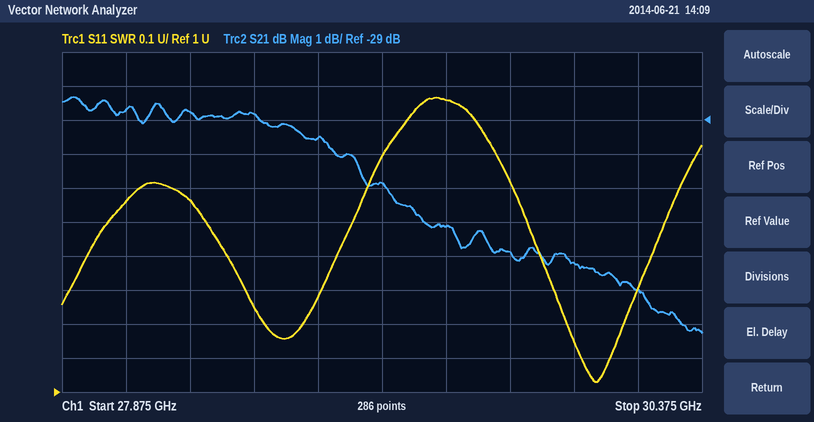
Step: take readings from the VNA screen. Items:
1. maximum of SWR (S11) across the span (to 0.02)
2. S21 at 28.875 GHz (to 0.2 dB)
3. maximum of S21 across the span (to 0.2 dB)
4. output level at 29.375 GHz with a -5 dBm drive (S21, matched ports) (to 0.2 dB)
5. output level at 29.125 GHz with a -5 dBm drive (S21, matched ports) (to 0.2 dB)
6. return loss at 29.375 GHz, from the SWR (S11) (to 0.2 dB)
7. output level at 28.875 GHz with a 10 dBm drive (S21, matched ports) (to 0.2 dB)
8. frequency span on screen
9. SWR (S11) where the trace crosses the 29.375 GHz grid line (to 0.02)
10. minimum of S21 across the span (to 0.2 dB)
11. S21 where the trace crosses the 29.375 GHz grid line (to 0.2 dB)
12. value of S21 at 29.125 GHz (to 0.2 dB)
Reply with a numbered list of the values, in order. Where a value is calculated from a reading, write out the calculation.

1. 1.86
2. -29.6 dB
3. -28.4 dB
4. -5 dBm + (-32.2 dB) = -37.2 dBm
5. -5 dBm + (-30.8 dB) = -35.8 dBm
6. −20 log10((1.86 − 1)/(1.86 + 1)) ≈ 10.4 dB
7. 10 dBm + (-29.6 dB) = -19.6 dBm
8. 2.5 GHz
9. 1.86
10. -35.2 dB
11. -32.2 dB
12. -30.8 dB
